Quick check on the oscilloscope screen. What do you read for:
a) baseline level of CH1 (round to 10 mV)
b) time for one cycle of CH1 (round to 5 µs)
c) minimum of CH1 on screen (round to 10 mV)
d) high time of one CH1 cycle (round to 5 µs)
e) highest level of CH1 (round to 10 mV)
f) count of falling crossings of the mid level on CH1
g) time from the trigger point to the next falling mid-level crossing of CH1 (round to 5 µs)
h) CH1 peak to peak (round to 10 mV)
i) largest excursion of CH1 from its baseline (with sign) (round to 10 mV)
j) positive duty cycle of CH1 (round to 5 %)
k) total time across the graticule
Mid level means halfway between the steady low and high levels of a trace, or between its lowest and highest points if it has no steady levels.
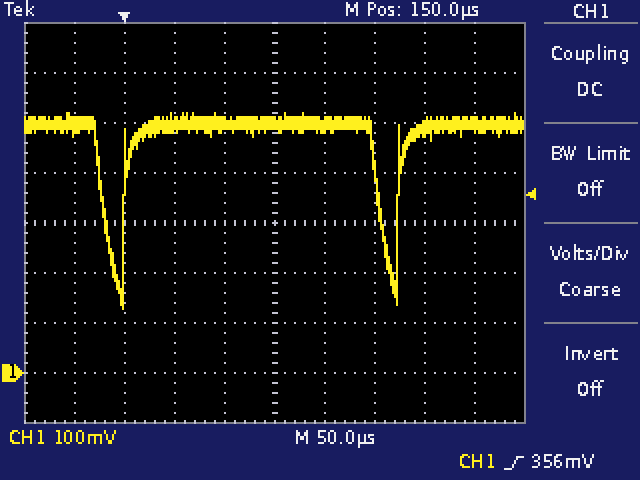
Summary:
500 mV
275 µs
130 mV
255 µs
520 mV
2
255 µs
390 mV
-370 mV
95 %
500 µs
